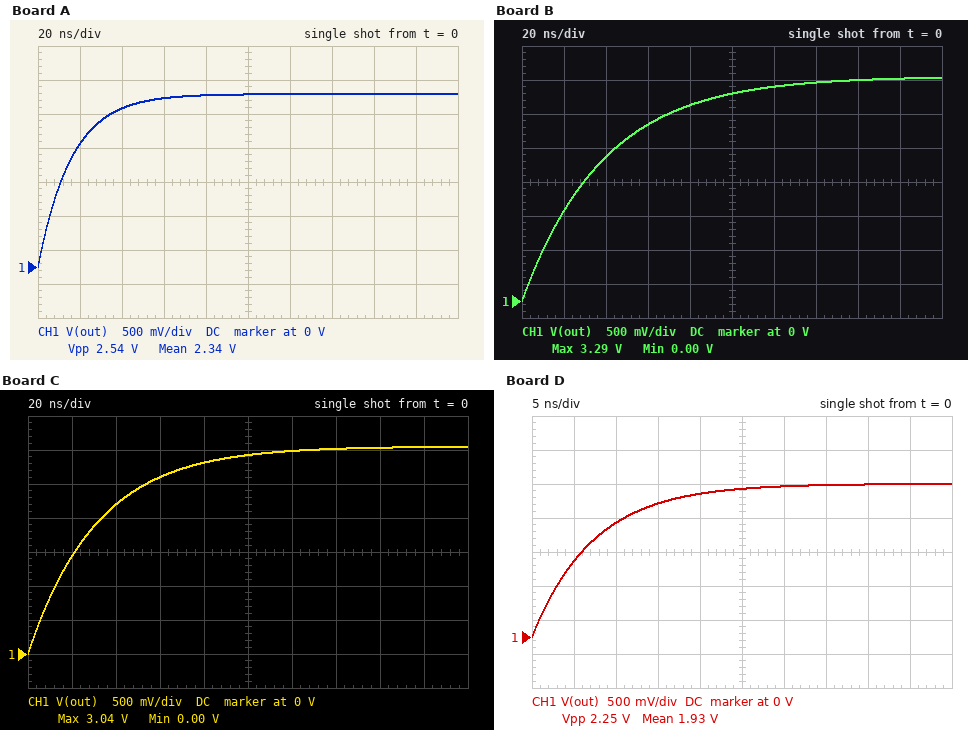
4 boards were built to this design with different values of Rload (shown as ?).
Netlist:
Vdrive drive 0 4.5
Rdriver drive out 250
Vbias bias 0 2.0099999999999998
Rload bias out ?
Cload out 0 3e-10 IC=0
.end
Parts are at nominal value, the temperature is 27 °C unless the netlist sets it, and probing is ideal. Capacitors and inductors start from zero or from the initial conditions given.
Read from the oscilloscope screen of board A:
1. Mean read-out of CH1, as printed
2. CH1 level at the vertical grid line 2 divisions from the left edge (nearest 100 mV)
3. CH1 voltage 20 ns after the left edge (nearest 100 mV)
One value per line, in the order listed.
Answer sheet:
2.34 V
2.3 V
1.8 V
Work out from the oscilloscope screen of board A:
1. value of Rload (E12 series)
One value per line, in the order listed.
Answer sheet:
68 Ω
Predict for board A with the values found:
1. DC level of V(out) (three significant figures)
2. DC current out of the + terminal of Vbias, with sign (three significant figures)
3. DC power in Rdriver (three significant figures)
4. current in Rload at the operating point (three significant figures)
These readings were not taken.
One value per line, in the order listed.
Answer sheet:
2.54 V
-7.83 mA
15.3 mW
7.83 mA
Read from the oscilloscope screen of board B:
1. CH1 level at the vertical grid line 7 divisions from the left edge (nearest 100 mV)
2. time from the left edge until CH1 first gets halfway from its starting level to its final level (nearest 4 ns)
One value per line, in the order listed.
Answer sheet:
3.2 V
28 ns
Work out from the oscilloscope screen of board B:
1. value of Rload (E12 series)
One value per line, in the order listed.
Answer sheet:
270 Ω
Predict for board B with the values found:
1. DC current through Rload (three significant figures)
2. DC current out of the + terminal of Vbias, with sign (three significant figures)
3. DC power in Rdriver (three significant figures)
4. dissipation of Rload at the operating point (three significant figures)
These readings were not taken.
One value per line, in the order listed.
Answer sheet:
4.79 mA
-4.79 mA
5.73 mW
6.19 mW
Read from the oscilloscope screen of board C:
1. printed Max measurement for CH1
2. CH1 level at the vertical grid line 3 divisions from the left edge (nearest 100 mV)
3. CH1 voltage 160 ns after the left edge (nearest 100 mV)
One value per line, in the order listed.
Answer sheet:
3.04 V
2.6 V
3.0 V
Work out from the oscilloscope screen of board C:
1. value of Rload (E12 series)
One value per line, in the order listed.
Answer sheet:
180 Ω
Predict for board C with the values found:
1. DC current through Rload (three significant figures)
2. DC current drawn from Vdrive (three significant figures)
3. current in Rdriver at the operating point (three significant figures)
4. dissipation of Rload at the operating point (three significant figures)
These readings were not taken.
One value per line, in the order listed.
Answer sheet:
5.79 mA
5.79 mA
5.79 mA
6.04 mW
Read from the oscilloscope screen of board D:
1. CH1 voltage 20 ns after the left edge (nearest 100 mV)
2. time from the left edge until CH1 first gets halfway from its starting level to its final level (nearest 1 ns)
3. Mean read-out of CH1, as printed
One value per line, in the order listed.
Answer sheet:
2.1 V
5 ns
1.93 V
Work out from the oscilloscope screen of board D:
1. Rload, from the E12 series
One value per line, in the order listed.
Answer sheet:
27 Ω
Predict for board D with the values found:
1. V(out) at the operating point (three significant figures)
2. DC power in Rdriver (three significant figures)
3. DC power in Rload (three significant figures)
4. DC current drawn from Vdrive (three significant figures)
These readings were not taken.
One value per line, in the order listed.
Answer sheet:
2.25 V
20.2 mW
2.18 mW
8.99 mA
